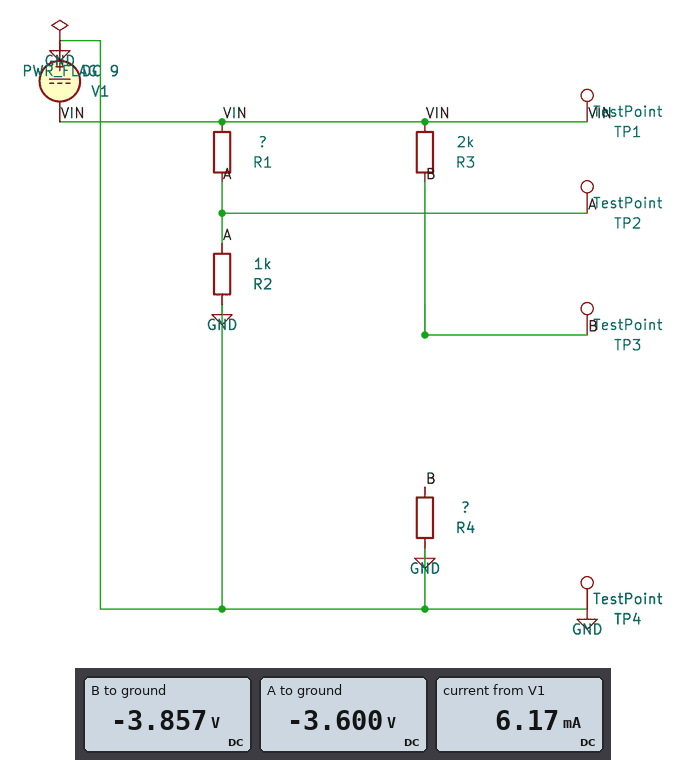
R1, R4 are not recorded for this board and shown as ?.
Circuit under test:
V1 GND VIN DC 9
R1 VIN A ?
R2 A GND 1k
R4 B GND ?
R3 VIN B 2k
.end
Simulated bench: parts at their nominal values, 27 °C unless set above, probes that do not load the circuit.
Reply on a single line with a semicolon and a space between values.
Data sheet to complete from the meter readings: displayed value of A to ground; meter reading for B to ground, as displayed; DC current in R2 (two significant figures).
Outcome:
-3.600 V; -3.857 V; 3.6 mA
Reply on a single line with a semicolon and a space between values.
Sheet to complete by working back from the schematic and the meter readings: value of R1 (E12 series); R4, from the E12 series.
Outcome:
1.5 kΩ; 1.5 kΩ
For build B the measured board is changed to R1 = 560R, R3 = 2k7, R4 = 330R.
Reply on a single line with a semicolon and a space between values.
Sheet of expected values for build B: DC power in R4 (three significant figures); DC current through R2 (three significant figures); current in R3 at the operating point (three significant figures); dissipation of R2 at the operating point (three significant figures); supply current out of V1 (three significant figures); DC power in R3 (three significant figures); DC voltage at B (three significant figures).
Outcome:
2.91 mW; 5.77 mA; 2.97 mA; 33.3 mW; 8.74 mA; 23.8 mW; -980 mV
